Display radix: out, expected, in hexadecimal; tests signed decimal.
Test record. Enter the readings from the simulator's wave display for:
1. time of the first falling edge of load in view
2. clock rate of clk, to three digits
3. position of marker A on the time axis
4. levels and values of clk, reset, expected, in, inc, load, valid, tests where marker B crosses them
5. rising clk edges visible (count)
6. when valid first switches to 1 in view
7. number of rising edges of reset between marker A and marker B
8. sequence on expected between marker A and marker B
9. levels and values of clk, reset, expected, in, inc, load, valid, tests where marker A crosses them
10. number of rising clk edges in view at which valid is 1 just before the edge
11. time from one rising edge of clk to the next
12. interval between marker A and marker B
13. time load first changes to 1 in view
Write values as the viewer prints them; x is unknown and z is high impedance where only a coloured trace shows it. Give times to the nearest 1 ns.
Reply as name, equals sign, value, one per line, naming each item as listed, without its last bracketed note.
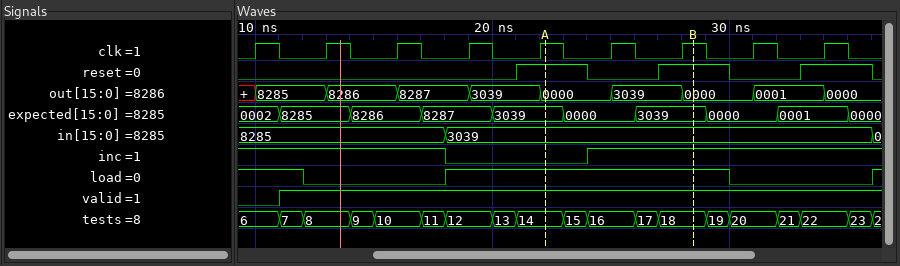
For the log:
time of the first falling edge of load in view = 12 ns
clock rate of clk, to three digits = 333 MHz
position of marker A on the time axis = 22 ns
levels and values of clk, reset, expected, in, inc, load, valid, tests where marker B crosses them = clk=1, reset=1, expected=3039, in=3039, inc=1, load=1, valid=1, tests=18
rising clk edges visible = 9
when valid first switches to 1 in view = 11 ns
number of rising edges of reset between marker A and marker B = 1
sequence on expected between marker A and marker B = 3039, 0000, 3039
levels and values of clk, reset, expected, in, inc, load, valid, tests where marker A crosses them = clk=1, reset=1, expected=3039, in=3039, inc=0, load=1, valid=1, tests=14
number of rising clk edges in view at which valid is 1 just before the edge = 8
time from one rising edge of clk to the next = 3 ns
interval between marker A and marker B = 6 ns
time load first changes to 1 in view = 18 ns
